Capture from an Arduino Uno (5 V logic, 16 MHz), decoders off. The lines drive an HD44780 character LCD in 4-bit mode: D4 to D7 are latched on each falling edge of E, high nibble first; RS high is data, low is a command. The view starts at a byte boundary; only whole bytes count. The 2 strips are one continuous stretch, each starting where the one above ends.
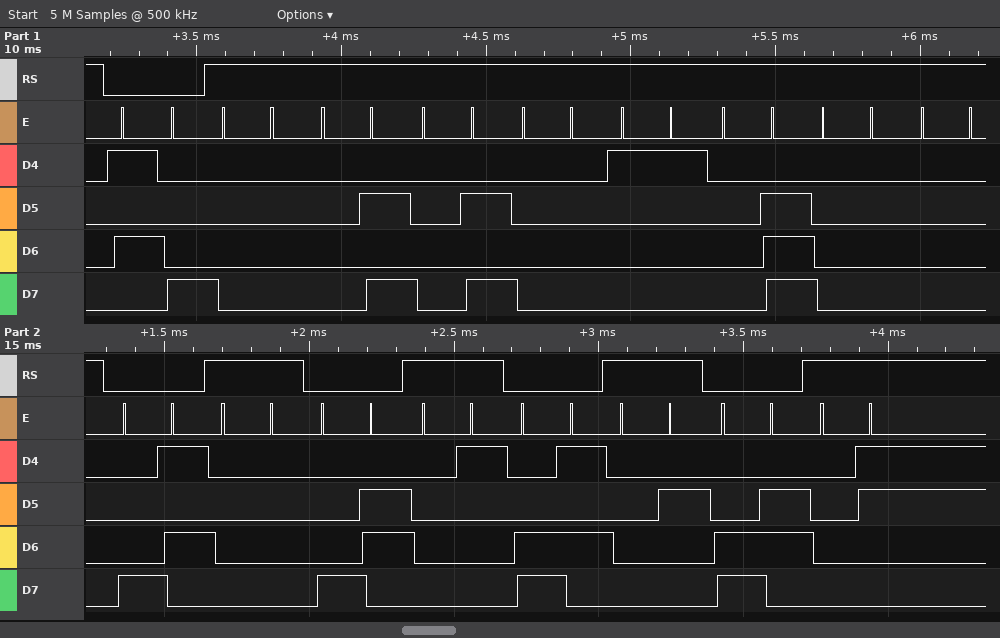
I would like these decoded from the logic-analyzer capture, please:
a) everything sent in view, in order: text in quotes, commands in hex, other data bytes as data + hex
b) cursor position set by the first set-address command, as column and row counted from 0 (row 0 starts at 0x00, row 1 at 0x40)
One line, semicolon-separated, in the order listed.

0x58 data 00 0A 0A 00 11 0E 00 00 0x85 data 00 0x86 data 01 0xC5 data 02 0xC6 data 03; column 5, row 0
